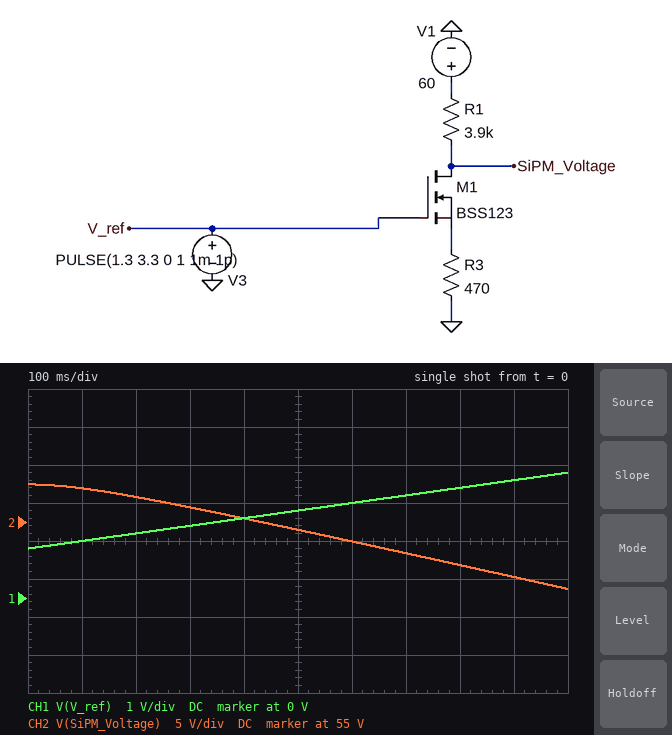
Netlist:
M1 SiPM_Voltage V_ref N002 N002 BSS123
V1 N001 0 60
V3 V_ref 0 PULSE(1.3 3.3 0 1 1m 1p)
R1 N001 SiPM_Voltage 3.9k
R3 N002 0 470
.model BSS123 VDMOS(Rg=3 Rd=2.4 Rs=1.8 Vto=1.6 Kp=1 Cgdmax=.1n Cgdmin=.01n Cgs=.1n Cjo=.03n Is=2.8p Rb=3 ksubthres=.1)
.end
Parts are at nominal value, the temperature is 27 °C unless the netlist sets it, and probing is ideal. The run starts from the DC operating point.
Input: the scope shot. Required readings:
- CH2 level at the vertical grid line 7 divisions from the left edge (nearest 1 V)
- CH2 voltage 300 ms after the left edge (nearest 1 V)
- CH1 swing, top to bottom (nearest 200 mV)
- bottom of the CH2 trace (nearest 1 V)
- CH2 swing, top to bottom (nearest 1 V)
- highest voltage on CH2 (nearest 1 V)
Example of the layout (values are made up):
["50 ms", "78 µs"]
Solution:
["51 V", "57 V", "2.0 V", "46 V", "14 V", "60 V"]
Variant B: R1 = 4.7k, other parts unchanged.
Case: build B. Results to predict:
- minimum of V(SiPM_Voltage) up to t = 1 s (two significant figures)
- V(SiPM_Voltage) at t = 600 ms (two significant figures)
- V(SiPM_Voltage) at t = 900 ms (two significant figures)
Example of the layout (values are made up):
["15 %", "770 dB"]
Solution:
["43 V", "51 V", "45 V"]
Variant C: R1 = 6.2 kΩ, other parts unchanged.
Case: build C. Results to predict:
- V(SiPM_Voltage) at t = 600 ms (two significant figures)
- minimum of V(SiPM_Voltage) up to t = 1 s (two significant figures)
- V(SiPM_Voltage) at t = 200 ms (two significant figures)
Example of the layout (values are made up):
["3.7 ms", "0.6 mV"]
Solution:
["48 V", "38 V", "57 V"]
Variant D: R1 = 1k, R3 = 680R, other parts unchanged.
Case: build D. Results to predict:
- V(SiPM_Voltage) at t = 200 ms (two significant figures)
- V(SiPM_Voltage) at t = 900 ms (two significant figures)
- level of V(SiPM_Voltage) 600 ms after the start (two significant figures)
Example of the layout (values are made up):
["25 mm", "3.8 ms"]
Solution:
["60 V", "58 V", "59 V"]
